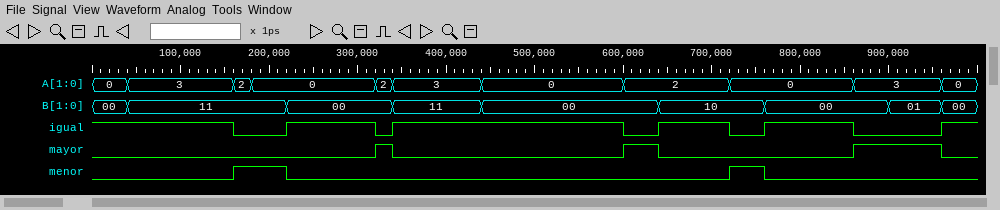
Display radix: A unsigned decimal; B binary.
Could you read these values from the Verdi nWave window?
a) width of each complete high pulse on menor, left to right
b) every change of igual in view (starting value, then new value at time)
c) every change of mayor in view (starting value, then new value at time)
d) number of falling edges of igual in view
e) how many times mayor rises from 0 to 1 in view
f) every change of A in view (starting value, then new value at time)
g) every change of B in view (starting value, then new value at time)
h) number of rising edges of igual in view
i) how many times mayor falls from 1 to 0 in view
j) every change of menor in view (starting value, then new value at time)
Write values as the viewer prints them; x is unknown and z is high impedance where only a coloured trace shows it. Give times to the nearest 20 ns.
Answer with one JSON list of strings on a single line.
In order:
["60 ns, 40 ns", "1, 0 at 160 ns, 1 at 220 ns, 0 at 320 ns, 1 at 340 ns, 0 at 600 ns, 1 at 640 ns, 0 at 720 ns, 1 at 760 ns, 0 at 860 ns, 1 at 960 ns", "0, 1 at 320 ns, 0 at 340 ns, 1 at 600 ns, 0 at 640 ns, 1 at 860 ns, 0 at 960 ns", "5", "3", "0, 3 at 40 ns, 2 at 160 ns, 0 at 180 ns, 2 at 320 ns, 3 at 340 ns, 0 at 440 ns, 2 at 600 ns, 0 at 720 ns, 3 at 860 ns, 0 at 960 ns", "00, 11 at 40 ns, 00 at 220 ns, 11 at 340 ns, 00 at 440 ns, 10 at 640 ns, 00 at 760 ns, 01 at 900 ns, 00 at 960 ns", "5", "3", "0, 1 at 160 ns, 0 at 220 ns, 1 at 720 ns, 0 at 760 ns"]
